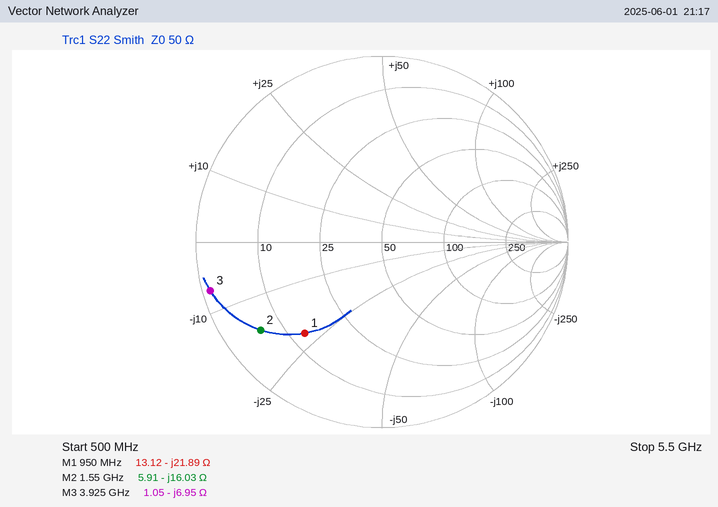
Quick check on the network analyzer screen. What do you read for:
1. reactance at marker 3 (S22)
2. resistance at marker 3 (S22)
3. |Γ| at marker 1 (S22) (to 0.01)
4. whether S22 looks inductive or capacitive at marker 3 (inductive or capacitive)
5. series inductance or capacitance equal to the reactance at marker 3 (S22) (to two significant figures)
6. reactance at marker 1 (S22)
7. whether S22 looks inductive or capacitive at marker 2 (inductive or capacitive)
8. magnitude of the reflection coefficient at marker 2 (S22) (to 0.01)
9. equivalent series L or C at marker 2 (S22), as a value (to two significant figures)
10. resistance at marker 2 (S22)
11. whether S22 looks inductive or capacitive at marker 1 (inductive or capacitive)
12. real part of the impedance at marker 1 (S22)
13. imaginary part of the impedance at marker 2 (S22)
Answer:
-6.95 Ω
1.05 Ω
0.64
capacitive
5.8 pF
-21.89 Ω
capacitive
0.81
6.4 pF
5.91 Ω
capacitive
13.12 Ω
-16.03 Ω
